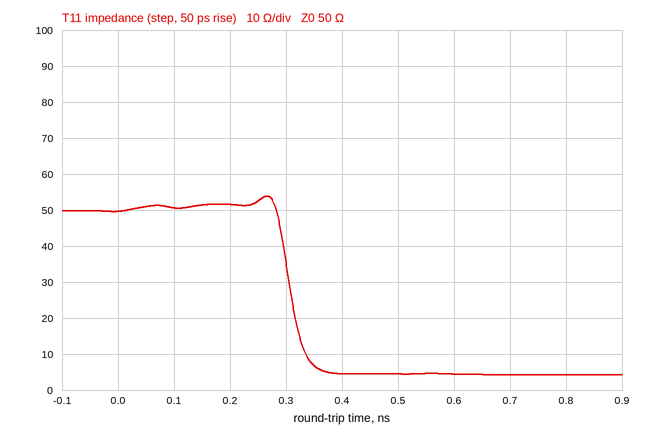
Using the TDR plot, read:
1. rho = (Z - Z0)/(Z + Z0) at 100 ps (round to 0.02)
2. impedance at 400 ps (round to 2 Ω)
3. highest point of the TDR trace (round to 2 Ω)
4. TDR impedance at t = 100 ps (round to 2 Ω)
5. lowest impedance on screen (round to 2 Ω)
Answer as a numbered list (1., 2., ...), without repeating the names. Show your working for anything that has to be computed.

1. (50 − 50)/(50 + 50) ≈ 0.00
2. 4 Ω
3. 54 Ω
4. 50 Ω
5. 4 Ω
